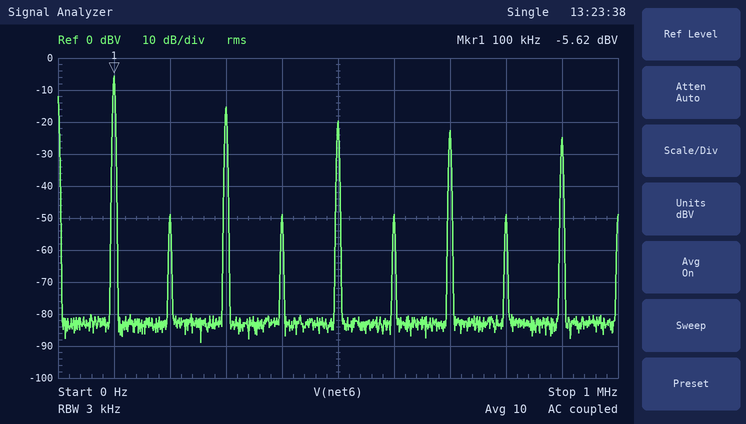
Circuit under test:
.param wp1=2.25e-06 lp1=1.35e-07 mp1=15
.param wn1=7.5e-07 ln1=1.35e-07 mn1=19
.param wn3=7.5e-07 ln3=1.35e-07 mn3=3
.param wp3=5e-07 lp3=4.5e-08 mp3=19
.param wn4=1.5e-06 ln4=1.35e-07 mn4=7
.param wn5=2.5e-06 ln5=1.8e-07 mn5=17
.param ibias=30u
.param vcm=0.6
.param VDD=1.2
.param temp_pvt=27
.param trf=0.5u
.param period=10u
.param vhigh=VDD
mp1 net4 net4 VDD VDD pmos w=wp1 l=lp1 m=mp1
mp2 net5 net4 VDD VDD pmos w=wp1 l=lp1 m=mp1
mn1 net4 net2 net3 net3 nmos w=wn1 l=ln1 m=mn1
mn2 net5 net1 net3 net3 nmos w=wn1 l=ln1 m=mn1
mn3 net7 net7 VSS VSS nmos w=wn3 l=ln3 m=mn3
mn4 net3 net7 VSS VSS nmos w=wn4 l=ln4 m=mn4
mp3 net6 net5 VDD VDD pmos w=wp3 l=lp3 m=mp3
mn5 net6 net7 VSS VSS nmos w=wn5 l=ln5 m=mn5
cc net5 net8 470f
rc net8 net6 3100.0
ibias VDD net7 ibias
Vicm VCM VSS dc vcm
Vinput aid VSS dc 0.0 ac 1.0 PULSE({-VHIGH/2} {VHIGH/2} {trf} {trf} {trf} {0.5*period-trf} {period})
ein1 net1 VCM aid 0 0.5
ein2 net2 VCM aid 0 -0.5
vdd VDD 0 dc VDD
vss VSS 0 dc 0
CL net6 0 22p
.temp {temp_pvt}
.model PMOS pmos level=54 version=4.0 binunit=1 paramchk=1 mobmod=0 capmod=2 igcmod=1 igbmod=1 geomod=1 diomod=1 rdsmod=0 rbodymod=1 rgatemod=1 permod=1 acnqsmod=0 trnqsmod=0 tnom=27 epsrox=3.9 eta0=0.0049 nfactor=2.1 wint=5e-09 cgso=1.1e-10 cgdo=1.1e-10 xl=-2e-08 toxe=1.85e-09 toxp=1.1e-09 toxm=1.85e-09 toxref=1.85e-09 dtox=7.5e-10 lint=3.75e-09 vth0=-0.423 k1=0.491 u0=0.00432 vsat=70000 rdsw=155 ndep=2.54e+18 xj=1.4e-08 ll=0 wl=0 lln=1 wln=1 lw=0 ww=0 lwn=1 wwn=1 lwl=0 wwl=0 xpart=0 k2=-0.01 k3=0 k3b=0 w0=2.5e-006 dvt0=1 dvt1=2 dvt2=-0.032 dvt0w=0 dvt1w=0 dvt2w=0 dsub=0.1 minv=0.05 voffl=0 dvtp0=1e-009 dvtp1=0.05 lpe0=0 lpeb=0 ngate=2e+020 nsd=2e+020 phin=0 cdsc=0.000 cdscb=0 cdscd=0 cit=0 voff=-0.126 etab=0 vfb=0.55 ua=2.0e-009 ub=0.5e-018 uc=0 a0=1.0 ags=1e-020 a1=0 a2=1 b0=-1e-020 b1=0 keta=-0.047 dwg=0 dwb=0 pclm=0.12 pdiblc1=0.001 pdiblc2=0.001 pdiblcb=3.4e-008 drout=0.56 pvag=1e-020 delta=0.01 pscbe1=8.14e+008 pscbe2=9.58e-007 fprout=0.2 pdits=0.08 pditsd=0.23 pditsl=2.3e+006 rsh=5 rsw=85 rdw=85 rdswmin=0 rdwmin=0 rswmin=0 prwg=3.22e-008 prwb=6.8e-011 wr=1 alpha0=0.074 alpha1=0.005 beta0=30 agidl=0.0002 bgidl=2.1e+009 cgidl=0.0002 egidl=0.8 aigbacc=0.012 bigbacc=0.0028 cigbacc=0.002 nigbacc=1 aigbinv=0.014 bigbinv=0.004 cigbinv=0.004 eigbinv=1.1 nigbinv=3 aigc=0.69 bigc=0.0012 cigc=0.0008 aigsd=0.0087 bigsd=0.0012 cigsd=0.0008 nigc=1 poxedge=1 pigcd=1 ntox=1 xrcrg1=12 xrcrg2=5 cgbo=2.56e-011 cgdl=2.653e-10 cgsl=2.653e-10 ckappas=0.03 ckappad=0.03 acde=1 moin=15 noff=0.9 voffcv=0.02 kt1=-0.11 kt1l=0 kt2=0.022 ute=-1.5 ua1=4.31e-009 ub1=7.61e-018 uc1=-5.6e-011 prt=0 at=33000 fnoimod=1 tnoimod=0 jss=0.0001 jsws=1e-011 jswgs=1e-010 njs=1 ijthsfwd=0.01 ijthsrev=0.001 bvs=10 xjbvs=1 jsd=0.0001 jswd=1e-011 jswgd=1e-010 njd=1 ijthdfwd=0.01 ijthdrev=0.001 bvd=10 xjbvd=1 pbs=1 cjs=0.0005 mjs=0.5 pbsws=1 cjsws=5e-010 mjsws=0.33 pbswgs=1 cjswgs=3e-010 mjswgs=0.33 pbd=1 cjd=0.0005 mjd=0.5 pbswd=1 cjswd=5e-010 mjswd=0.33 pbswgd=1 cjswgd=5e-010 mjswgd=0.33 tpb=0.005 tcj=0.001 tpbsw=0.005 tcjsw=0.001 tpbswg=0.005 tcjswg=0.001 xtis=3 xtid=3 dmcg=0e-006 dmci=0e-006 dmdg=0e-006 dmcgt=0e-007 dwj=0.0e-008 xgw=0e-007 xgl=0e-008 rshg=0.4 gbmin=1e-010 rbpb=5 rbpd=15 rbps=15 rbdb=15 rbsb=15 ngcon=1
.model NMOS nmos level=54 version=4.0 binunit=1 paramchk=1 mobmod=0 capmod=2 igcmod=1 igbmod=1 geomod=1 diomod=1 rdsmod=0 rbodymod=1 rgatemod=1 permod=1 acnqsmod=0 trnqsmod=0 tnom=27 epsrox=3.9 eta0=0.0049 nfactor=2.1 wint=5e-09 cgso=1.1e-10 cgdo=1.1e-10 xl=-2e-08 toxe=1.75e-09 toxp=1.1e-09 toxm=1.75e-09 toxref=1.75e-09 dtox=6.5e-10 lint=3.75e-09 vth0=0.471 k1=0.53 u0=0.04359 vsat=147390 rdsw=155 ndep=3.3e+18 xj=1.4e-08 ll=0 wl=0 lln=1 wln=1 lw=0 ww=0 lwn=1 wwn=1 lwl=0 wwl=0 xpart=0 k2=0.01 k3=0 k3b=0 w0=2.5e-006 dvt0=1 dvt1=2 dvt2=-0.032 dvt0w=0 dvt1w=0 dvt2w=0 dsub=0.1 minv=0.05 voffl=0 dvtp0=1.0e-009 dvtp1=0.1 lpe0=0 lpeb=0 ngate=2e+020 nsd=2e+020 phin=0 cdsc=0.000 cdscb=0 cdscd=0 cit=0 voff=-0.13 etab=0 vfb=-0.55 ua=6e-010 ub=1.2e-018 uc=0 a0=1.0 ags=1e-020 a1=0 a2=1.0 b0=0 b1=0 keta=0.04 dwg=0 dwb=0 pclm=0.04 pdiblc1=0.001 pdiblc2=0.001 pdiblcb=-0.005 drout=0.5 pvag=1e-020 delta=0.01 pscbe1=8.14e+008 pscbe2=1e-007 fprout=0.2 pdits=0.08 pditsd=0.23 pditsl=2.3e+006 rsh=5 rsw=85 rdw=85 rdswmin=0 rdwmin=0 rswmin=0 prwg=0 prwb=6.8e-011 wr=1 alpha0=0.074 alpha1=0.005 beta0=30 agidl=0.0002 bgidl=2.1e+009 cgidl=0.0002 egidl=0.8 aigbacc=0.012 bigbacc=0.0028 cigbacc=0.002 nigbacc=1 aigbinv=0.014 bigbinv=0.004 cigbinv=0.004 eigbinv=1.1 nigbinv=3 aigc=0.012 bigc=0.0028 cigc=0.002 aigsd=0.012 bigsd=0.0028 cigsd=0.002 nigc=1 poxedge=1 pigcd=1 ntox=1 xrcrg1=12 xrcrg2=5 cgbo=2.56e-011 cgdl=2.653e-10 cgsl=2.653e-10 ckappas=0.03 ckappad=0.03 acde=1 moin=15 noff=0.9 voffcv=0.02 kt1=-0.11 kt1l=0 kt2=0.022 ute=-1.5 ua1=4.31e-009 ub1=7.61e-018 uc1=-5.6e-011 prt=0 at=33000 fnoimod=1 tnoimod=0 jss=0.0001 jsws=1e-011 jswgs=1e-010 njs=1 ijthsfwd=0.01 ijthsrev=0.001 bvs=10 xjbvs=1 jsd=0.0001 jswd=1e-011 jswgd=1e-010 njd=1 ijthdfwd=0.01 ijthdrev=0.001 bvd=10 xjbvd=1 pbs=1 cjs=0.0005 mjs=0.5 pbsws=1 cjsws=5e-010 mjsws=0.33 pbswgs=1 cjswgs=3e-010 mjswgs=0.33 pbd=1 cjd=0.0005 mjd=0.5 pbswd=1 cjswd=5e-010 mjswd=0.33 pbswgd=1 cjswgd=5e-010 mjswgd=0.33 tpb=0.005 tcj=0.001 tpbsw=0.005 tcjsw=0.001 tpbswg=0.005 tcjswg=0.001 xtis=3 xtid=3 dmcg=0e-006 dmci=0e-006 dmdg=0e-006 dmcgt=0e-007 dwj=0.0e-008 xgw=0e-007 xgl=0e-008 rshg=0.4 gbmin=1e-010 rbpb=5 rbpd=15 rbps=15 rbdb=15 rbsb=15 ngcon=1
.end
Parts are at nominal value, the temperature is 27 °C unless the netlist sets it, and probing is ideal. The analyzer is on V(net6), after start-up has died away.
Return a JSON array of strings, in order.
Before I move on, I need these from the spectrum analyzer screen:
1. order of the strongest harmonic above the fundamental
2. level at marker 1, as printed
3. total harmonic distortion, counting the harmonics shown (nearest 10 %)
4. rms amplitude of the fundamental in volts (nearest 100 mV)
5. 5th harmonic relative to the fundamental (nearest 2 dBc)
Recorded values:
["3", "-5.62 dBV", "40 %", "500 mV", "-14 dBc"]
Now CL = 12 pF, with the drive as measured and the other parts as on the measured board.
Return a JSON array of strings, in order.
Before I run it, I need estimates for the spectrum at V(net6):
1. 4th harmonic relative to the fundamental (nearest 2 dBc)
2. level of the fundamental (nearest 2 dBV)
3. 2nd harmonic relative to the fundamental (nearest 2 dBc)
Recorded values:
["-50 dBc", "-6 dBV", "-50 dBc"]
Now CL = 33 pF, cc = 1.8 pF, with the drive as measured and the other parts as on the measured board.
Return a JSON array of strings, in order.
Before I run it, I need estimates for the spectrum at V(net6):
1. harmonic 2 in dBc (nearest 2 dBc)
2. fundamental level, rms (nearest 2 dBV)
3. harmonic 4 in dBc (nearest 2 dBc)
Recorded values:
["-40 dBc", "-6 dBV", "-40 dBc"]
